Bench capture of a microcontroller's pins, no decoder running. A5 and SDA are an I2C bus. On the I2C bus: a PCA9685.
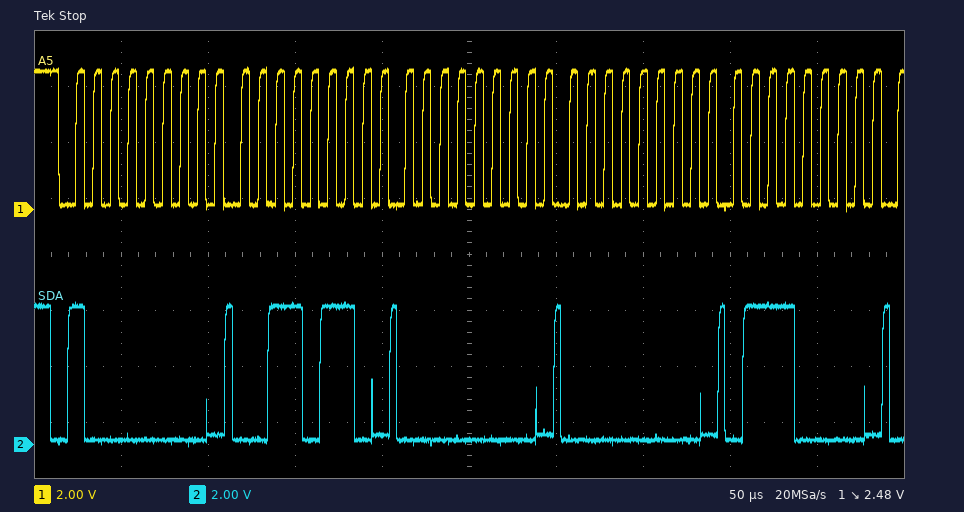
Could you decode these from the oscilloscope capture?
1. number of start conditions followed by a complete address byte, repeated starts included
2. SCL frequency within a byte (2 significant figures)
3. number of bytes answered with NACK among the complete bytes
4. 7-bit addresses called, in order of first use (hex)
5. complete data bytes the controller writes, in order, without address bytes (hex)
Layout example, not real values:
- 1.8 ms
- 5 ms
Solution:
- 1
- 100 kHz
- 0
- 0x40
- 36 00 00 70
